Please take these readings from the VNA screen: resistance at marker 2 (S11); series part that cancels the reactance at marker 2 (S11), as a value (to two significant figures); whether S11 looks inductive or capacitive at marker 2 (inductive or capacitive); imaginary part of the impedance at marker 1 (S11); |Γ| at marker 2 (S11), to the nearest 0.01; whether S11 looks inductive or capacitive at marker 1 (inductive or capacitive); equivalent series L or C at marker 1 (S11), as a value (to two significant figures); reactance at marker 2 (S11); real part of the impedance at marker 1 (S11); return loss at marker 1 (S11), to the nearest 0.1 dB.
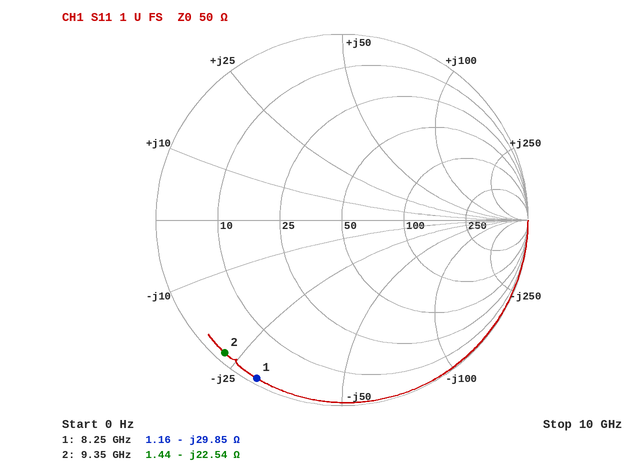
1.44 Ω
380 pH
capacitive
-29.85 Ω
0.95
capacitive
650 fF
-22.54 Ω
1.16 Ω
0.3 dB
